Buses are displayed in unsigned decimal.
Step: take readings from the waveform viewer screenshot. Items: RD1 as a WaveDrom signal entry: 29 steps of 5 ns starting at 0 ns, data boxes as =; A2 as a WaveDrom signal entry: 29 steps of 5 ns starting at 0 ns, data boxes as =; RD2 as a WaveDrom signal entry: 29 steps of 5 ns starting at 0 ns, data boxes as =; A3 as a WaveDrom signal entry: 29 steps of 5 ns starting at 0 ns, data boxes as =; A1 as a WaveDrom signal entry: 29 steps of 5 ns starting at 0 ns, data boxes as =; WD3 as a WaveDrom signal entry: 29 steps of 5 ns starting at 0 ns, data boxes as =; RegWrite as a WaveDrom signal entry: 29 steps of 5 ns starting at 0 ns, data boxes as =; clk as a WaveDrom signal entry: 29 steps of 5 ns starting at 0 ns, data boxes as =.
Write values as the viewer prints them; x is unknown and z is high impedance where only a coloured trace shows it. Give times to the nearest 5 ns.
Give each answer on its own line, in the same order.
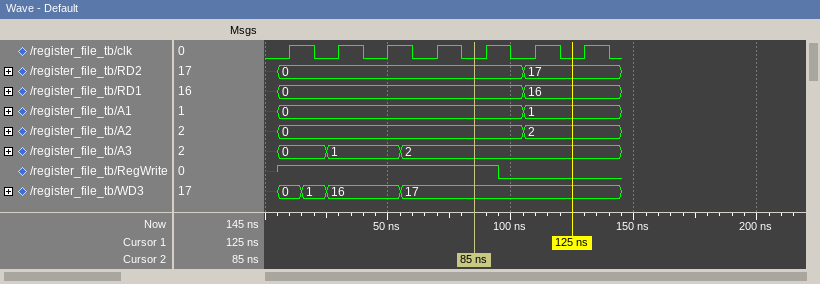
{name: 'RD1', wave: 'x=...................=.......', data: '0 16'}
{name: 'A2', wave: 'x=...................=.......', data: '0 2'}
{name: 'RD2', wave: 'x=...................=.......', data: '0 17'}
{name: 'A3', wave: 'x=...=.....=.................', data: '0 1 2'}
{name: 'A1', wave: 'x=...................=.......', data: '0 1'}
{name: 'WD3', wave: 'x=.=.=.....=.................', data: '0 1 16 17'}
{name: 'RegWrite', wave: 'x1.................0.........'}
{name: 'clk', wave: '0.1.0.1.0.1.0.1.0.1.0.1.0.1.0'}
